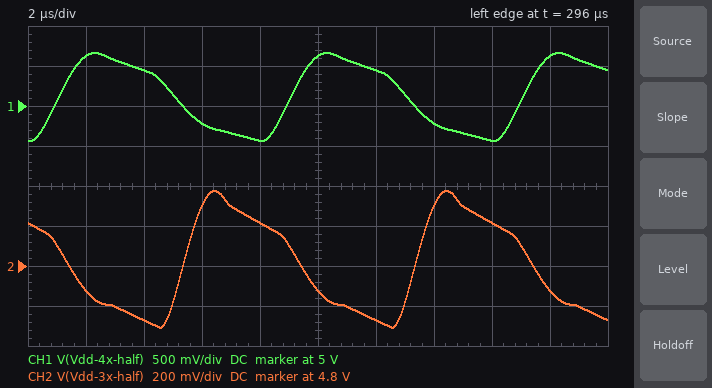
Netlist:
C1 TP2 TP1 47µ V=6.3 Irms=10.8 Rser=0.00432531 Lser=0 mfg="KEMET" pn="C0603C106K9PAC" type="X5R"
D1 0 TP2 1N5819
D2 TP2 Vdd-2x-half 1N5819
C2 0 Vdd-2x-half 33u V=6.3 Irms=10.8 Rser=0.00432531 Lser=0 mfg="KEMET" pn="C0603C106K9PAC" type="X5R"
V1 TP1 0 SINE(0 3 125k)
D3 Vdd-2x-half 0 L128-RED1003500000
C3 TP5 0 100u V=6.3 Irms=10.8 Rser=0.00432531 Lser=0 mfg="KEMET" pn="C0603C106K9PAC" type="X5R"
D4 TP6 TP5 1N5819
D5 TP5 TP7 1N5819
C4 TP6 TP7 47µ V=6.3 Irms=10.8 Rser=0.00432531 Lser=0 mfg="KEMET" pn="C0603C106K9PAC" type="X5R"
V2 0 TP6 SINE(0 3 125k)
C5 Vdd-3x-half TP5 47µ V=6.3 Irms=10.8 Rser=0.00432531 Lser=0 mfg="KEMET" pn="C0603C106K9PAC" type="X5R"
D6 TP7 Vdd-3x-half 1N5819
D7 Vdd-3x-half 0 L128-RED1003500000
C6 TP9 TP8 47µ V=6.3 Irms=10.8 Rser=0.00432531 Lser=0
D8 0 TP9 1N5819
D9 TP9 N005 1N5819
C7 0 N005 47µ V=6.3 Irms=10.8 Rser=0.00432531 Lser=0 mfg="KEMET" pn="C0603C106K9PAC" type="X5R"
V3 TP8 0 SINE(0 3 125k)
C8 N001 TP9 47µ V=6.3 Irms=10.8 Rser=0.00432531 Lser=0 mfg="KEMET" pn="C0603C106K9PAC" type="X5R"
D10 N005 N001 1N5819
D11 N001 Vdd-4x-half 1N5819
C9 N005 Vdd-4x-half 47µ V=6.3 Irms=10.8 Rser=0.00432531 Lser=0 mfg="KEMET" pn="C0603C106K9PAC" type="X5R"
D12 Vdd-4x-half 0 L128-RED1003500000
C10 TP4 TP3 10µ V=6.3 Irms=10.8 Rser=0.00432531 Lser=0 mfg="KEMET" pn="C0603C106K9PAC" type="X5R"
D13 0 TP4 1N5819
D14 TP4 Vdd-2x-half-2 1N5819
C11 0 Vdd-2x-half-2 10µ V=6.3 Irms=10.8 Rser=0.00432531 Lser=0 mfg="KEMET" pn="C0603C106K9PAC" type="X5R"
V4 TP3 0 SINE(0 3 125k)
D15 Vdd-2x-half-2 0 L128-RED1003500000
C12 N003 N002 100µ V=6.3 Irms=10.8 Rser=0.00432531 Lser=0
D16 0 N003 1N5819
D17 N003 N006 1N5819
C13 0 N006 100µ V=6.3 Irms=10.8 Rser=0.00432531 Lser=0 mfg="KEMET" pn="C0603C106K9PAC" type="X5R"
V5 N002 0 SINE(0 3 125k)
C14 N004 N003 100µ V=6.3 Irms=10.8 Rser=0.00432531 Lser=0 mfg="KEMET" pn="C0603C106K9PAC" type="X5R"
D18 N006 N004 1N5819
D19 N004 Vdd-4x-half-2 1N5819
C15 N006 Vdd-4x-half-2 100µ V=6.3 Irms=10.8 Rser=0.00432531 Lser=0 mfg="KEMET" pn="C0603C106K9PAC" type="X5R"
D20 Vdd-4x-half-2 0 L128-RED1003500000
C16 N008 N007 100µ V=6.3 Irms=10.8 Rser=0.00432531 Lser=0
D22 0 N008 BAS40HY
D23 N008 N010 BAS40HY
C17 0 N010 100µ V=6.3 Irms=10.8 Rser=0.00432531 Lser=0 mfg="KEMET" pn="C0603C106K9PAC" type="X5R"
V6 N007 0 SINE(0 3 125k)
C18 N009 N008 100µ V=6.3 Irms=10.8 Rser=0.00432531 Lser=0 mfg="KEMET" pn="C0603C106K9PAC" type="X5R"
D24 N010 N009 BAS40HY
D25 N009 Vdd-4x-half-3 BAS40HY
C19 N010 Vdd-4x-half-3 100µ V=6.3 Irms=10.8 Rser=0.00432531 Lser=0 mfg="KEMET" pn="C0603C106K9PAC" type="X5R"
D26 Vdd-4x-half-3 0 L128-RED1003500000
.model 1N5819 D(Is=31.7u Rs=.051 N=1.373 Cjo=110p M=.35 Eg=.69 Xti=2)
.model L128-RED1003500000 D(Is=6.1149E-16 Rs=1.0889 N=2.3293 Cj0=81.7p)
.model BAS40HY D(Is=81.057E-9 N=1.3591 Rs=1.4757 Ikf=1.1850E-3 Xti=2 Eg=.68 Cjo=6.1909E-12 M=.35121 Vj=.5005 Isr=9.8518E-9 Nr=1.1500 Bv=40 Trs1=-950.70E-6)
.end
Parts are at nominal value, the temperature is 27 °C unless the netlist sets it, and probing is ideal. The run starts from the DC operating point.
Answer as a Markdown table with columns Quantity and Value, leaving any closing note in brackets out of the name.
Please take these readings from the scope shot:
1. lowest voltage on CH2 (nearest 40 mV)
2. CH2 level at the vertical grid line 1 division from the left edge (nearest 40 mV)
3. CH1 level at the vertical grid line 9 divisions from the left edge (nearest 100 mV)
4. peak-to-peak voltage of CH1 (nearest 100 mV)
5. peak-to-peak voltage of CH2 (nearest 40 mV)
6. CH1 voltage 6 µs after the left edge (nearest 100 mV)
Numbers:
| Quantity | Value |
|---|---|
| lowest voltage on CH2 | 4.48 V |
| CH2 level at the vertical grid line 1 division from the left edge | 4.68 V |
| CH1 level at the vertical grid line 9 divisions from the left edge | 5.6 V |
| peak-to-peak voltage of CH1 | 1.1 V |
| peak-to-peak voltage of CH2 | 680 mV |
| CH1 voltage 6 µs after the left edge | 4.8 V |
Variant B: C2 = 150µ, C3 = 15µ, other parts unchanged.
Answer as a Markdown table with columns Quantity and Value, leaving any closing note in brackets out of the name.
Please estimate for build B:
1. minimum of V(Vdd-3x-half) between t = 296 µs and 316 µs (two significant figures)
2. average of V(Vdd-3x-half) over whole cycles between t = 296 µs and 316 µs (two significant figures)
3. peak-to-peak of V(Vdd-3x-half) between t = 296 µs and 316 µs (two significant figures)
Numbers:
| Quantity | Value |
|---|---|
| minimum of V(Vdd-3x-half) between t = 296 µs and 316 µs | 3.3 V |
| average of V(Vdd-3x-half) over whole cycles between t = 296 µs and 316 µs | 4.2 V |
| peak-to-peak of V(Vdd-3x-half) between t = 296 µs and 316 µs | 1.9 V |
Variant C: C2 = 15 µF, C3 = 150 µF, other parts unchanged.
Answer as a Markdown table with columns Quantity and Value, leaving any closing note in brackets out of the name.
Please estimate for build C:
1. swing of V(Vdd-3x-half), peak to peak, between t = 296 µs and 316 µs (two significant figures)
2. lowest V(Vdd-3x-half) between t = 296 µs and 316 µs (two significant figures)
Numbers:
| Quantity | Value |
|---|---|
| swing of V(Vdd-3x-half), peak to peak, between t = 296 µs and 316 µs | 590 mV |
| lowest V(Vdd-3x-half) between t = 296 µs and 316 µs | 4.6 V |
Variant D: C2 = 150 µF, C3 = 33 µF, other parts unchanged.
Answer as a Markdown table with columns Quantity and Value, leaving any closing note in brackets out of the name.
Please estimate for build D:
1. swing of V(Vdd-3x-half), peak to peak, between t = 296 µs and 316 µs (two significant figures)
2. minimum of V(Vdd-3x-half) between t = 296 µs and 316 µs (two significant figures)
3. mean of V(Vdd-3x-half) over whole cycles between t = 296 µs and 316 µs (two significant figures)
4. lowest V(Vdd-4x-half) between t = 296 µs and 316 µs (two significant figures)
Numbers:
| Quantity | Value |
|---|---|
| swing of V(Vdd-3x-half), peak to peak, between t = 296 µs and 316 µs | 1.2 V |
| minimum of V(Vdd-3x-half) between t = 296 µs and 316 µs | 4.0 V |
| mean of V(Vdd-3x-half) over whole cycles between t = 296 µs and 316 µs | 4.6 V |
| lowest V(Vdd-4x-half) between t = 296 µs and 316 µs | 4.6 V |
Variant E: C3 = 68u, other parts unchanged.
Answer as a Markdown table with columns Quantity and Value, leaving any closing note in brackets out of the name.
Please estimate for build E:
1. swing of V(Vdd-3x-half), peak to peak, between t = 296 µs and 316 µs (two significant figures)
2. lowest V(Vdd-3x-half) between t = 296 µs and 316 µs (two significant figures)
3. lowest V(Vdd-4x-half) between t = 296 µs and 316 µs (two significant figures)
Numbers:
| Quantity | Value |
|---|---|
| swing of V(Vdd-3x-half), peak to peak, between t = 296 µs and 316 µs | 820 mV |
| lowest V(Vdd-3x-half) between t = 296 µs and 316 µs | 4.4 V |
| lowest V(Vdd-4x-half) between t = 296 µs and 316 µs | 4.6 V |
